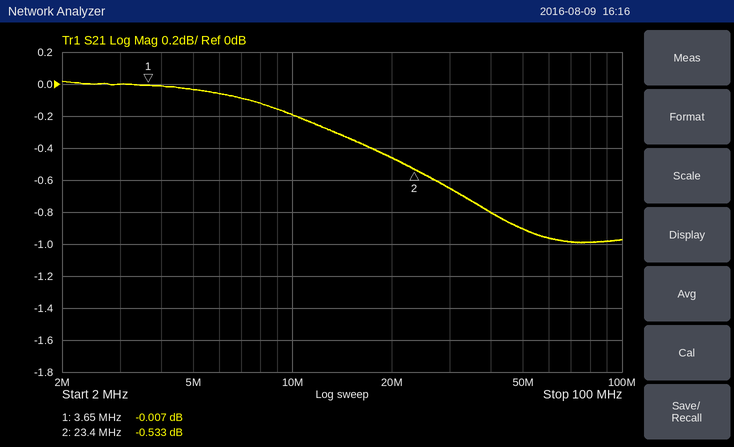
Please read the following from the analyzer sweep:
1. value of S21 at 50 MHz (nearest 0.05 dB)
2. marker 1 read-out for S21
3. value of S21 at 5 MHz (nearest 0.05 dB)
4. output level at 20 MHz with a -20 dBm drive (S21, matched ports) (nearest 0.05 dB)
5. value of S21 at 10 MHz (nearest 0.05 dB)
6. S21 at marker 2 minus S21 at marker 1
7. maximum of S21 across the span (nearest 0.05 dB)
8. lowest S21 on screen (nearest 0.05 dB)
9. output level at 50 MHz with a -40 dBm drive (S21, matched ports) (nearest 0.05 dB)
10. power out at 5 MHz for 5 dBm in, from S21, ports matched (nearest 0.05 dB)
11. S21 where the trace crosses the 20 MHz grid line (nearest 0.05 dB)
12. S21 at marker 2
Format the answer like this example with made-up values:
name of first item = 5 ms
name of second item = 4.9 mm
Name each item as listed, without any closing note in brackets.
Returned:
value of S21 at 50 MHz = -0.90 dB
marker 1 read-out for S21 = -0.007 dB
value of S21 at 5 MHz = -0.05 dB
output level at 20 MHz with a -20 dBm drive (S21, matched ports) = -20.45 dBm
value of S21 at 10 MHz = -0.20 dB
S21 at marker 2 minus S21 at marker 1 = -0.526 dB
maximum of S21 across the span = 0.00 dB
lowest S21 on screen = -1.00 dB
output level at 50 MHz with a -40 dBm drive (S21, matched ports) = -40.90 dBm
power out at 5 MHz for 5 dBm in, from S21, ports matched = 4.95 dBm
S21 where the trace crosses the 20 MHz grid line = -0.45 dB
S21 at marker 2 = -0.533 dB
